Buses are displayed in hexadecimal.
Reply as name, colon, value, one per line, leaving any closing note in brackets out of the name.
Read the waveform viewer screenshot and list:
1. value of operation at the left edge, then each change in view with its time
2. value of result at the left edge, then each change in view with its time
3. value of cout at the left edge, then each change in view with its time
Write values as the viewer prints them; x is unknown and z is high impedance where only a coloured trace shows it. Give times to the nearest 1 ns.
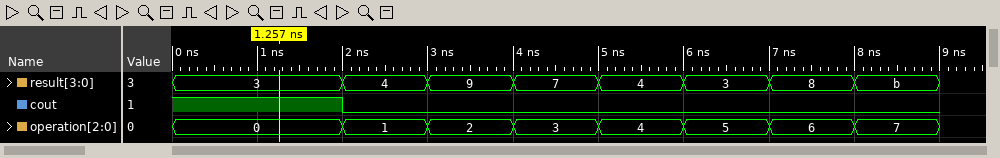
value of operation at the left edge, then each change in view with its time: 0, 1 at 2 ns, 2 at 3 ns, 3 at 4 ns, 4 at 5 ns, 5 at 6 ns, 6 at 7 ns, 7 at 8 ns
value of result at the left edge, then each change in view with its time: 3, 4 at 2 ns, 9 at 3 ns, 7 at 4 ns, 4 at 5 ns, 3 at 6 ns, 8 at 7 ns, b at 8 ns
value of cout at the left edge, then each change in view with its time: 1, 0 at 2 ns
